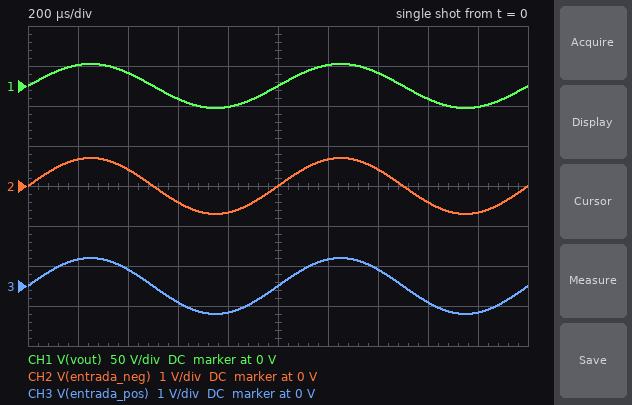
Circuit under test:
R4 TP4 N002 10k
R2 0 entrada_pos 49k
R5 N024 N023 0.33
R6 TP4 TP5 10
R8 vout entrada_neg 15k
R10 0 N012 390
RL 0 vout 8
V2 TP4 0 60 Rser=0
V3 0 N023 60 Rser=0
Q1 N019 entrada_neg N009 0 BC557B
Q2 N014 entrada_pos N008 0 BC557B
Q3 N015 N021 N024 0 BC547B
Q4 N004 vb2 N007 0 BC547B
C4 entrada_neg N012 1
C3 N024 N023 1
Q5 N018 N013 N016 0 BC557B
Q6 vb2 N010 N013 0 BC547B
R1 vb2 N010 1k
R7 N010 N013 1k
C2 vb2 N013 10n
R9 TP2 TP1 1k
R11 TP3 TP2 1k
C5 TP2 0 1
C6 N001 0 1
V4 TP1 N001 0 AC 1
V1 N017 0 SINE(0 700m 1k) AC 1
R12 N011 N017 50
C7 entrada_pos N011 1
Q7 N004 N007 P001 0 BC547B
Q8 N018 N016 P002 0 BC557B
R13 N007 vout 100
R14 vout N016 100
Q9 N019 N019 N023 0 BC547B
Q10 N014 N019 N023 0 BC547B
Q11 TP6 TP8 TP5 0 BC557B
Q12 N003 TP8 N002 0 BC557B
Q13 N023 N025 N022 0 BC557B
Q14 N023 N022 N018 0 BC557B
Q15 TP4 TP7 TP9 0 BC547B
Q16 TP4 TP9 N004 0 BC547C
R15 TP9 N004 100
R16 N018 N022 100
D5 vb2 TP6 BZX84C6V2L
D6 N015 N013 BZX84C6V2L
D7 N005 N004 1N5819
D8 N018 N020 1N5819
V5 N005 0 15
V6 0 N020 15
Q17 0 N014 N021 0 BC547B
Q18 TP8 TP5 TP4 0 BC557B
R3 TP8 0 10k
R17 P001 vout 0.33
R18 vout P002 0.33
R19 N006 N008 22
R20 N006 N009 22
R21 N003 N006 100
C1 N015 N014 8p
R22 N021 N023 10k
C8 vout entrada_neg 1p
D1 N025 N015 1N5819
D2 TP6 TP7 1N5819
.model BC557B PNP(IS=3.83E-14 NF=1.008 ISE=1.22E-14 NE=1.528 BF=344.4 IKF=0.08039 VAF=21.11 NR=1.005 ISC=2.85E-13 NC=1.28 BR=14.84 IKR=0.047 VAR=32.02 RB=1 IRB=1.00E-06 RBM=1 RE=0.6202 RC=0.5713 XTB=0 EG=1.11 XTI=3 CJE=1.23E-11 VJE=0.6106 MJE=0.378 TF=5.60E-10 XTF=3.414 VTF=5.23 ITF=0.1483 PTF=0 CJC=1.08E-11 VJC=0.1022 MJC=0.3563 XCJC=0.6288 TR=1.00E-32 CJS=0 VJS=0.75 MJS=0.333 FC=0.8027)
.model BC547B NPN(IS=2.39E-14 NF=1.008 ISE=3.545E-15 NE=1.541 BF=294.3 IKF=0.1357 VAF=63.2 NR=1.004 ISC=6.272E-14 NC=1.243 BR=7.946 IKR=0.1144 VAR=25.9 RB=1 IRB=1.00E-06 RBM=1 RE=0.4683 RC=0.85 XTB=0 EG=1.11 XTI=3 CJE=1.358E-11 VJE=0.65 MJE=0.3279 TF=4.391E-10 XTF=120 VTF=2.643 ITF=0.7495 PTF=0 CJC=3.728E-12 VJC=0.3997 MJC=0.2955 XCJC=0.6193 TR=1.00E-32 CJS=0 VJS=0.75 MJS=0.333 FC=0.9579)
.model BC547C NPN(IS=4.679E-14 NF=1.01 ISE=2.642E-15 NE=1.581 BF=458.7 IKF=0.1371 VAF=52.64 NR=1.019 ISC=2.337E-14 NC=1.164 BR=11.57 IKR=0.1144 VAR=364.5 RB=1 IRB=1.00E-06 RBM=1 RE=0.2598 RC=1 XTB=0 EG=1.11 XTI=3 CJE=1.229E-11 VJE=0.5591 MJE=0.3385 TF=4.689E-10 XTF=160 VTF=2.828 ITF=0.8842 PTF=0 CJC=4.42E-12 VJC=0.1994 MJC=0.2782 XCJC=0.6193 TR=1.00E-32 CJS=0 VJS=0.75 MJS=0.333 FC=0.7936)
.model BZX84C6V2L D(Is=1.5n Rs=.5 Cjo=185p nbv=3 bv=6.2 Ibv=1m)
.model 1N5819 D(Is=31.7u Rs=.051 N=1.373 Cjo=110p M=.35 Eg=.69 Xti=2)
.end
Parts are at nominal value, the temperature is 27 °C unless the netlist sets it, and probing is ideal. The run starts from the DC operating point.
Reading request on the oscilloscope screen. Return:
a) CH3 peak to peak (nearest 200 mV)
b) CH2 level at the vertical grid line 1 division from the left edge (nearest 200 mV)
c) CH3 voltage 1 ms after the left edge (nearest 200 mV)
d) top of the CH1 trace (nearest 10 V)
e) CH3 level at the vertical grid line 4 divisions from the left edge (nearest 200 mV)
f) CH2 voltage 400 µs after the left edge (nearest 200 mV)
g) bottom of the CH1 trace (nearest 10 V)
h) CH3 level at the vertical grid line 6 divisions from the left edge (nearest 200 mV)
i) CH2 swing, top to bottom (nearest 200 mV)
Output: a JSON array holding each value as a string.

["1.4 V", "600 mV", "0 V", "30 V", "-600 mV", "400 mV", "-30 V", "600 mV", "1.4 V"]
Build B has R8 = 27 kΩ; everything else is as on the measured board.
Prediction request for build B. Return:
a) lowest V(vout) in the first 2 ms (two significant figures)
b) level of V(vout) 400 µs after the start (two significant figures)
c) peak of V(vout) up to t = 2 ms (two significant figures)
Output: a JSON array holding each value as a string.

["-45 V", "29 V", "45 V"]
